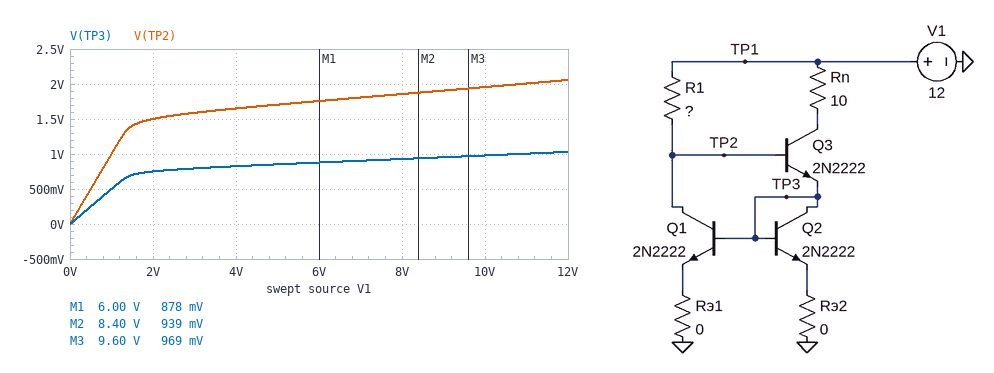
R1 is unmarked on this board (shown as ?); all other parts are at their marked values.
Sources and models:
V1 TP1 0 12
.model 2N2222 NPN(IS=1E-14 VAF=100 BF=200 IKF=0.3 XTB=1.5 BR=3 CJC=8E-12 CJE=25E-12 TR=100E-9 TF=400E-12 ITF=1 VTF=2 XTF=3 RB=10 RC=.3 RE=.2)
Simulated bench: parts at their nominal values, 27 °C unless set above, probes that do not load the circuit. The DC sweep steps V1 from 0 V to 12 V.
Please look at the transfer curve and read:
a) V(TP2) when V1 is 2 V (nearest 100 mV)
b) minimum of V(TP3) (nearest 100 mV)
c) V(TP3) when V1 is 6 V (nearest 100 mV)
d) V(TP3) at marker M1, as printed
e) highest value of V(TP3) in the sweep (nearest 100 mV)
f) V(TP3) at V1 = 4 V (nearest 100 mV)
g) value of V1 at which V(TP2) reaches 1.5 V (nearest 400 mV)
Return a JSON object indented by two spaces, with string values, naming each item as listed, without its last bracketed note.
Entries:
{
  "V(TP2) when V1 is 2 V": "1.5 V",
  "minimum of V(TP3)": "0 V",
  "V(TP3) when V1 is 6 V": "900 mV",
  "V(TP3) at marker M1, as printed": "878 mV",
  "highest value of V(TP3) in the sweep": "1.0 V",
  "V(TP3) at V1 = 4 V": "800 mV",
  "value of V1 at which V(TP2) reaches 1.5 V": "2.0 V"
}
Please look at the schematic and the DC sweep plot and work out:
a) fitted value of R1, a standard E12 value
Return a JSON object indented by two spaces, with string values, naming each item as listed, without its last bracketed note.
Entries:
{
  "fitted value of R1, a standard E12 value": "18 Ω"
}
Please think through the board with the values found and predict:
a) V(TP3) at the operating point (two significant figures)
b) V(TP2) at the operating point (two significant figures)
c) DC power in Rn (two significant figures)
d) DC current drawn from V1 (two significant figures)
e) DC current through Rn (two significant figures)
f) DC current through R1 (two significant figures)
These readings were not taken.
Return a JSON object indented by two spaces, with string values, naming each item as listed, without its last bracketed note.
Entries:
{
  "V(TP3) at the operating point": "1.0 V",
  "V(TP2) at the operating point": "2.1 V",
  "DC power in Rn": "3.0 W",
  "DC current drawn from V1": "1.1 A",
  "DC current through Rn": "550 mA",
  "DC current through R1": "550 mA"
}
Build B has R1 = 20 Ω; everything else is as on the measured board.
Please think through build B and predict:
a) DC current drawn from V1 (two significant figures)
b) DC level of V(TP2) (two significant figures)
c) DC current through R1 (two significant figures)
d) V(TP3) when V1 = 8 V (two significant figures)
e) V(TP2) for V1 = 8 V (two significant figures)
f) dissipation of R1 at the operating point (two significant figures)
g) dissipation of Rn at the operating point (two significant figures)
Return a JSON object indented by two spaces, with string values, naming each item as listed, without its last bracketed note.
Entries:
{
  "DC current drawn from V1": "1.0 A",
  "DC level of V(TP2)": "2.0 V",
  "DC current through R1": "500 mA",
  "V(TP3) when V1 = 8 V": "910 mV",
  "V(TP2) for V1 = 8 V": "1.8 V",
  "dissipation of R1 at the operating point": "5.0 W",
  "dissipation of Rn at the operating point": "2.5 W"
}
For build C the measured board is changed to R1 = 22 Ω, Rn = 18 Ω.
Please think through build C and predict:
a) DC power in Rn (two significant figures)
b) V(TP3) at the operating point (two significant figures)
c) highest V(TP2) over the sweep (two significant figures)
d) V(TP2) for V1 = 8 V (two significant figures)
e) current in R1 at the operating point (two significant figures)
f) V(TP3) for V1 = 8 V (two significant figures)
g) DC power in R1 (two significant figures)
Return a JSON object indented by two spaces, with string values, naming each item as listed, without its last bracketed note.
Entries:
{
  "DC power in Rn": "3.7 W",
  "V(TP3) at the operating point": "980 mV",
  "highest V(TP2) over the sweep": "2.0 V",
  "V(TP2) for V1 = 8 V": "1.8 V",
  "current in R1 at the operating point": "460 mA",
  "V(TP3) for V1 = 8 V": "900 mV",
  "DC power in R1": "4.6 W"
}
